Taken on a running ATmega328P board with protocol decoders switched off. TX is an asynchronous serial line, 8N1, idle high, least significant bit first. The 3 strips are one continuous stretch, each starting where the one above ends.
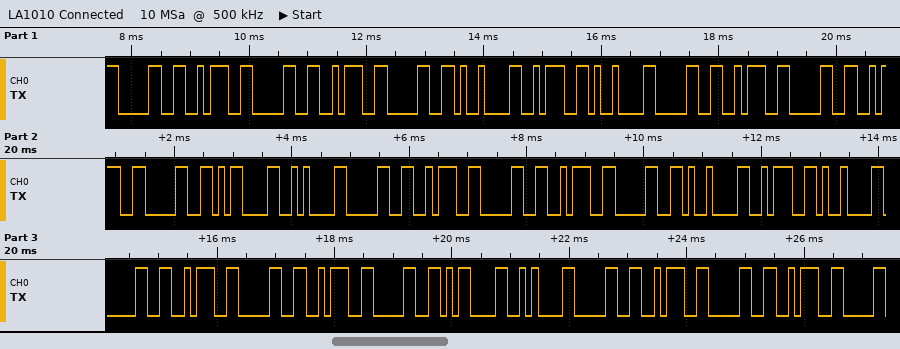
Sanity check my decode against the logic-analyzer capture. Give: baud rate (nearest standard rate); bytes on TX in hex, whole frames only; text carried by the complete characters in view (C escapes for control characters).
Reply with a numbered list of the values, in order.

1. 9600 baud
2. 30 3A 30 3A 30 09 3A 09 30 3A 30 3A 30 0D 0A 30 3A 30 3A 30 09 3A 09 30 3A 30 3A 30 0D 0A 30 3A 30 3A
3. "0:0:0\t:\t0:0:0\r\n0:0:0\t:\t0:0:0\r\n0:0:"
